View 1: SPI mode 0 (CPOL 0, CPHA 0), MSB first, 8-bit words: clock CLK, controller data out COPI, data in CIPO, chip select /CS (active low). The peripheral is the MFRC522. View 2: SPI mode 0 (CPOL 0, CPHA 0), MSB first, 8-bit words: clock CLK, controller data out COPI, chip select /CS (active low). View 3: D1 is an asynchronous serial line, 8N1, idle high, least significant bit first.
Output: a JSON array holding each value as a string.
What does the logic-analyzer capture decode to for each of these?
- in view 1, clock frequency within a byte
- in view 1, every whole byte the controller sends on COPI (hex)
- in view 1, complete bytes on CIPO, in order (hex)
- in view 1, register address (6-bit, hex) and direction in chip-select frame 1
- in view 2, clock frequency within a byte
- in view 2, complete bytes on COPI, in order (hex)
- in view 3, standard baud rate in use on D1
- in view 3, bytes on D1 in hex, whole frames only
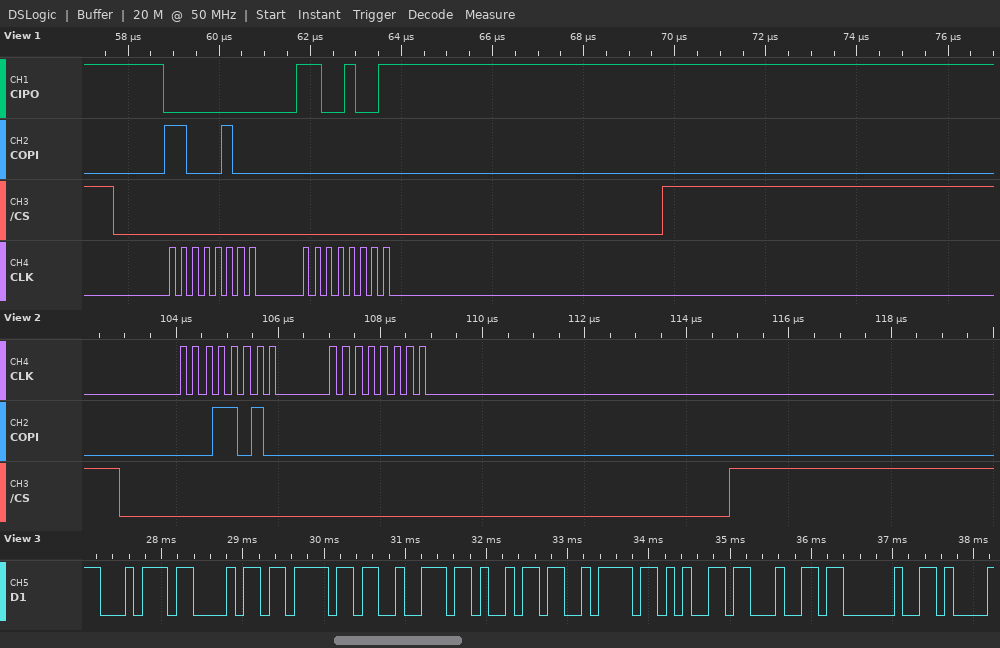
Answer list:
["4 MHz", "C4 00", "00 C9", "0x22 read", "4 MHz", "1A 00", "9600 baud", "74 68 6F 72 69 7A 65 64 20"]
